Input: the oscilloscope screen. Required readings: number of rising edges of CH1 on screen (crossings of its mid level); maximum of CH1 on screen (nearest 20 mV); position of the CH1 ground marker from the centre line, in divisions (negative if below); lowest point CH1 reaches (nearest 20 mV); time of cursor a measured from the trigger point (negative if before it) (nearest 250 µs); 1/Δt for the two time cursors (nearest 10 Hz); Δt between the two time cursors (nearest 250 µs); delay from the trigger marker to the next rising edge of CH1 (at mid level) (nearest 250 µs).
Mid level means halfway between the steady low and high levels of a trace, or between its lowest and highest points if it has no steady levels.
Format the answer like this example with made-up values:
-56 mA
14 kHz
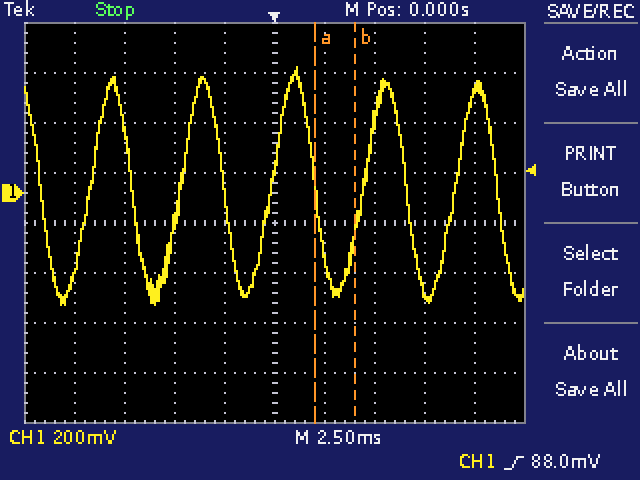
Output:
5
500 mV
+0.6 div
-440 mV
+2.00 ms
500 Hz
2.00 ms
4.50 ms
